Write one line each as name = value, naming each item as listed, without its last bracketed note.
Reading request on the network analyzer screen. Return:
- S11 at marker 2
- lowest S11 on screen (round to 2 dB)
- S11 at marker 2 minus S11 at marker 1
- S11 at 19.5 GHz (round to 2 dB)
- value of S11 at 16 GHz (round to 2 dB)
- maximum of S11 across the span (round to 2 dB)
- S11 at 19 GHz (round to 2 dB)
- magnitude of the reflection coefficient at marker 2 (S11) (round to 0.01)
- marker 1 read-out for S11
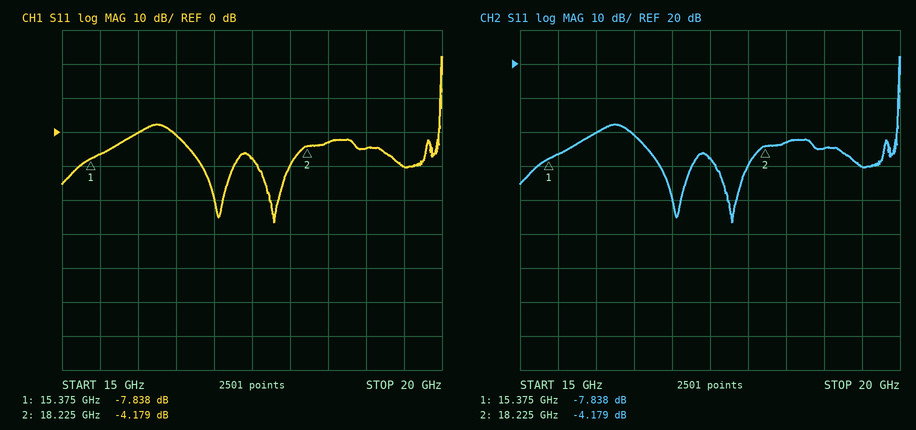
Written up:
S11 at marker 2 = -4.179 dB
lowest S11 on screen = -26 dB
S11 at marker 2 minus S11 at marker 1 = 3.659 dB
S11 at 19.5 GHz = -10 dB
value of S11 at 16 GHz = 0 dB
maximum of S11 across the span = 22 dB
S11 at 19 GHz = -4 dB
magnitude of the reflection coefficient at marker 2 (S11) = 0.62
marker 1 read-out for S11 = -7.838 dB
